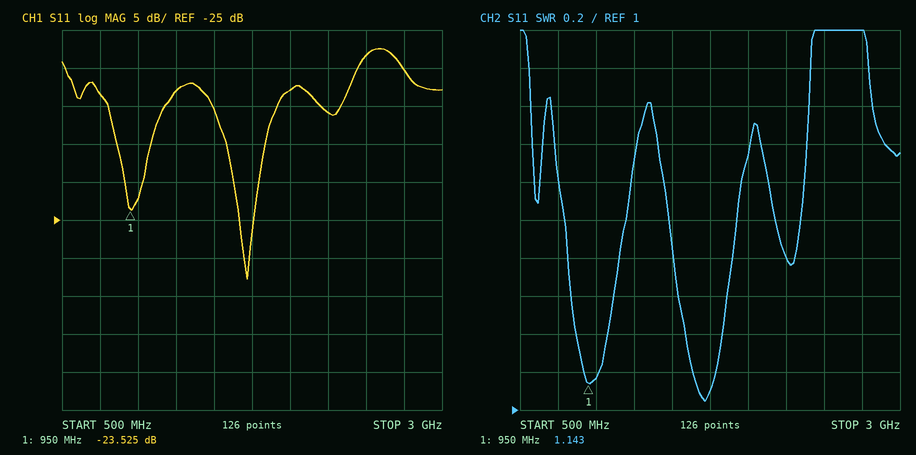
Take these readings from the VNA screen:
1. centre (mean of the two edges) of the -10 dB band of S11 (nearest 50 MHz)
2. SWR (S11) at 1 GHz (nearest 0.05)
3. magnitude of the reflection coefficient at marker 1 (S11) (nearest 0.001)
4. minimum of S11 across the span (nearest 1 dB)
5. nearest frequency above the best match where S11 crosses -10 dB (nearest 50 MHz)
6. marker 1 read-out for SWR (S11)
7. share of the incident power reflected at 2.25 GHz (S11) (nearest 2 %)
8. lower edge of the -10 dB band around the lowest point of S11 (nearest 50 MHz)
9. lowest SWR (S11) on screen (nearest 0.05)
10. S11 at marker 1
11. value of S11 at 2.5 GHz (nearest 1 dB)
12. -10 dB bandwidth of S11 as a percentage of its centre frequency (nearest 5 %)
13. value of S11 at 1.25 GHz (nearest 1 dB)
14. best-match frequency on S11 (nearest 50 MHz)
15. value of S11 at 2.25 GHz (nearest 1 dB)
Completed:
1.70 GHz
1.15
0.067
-33 dB
1.90 GHz
1.143
8 %
1.50 GHz
1.05
-23.525 dB
-3 dB
25 %
-8 dB
1.70 GHz
-11 dB
